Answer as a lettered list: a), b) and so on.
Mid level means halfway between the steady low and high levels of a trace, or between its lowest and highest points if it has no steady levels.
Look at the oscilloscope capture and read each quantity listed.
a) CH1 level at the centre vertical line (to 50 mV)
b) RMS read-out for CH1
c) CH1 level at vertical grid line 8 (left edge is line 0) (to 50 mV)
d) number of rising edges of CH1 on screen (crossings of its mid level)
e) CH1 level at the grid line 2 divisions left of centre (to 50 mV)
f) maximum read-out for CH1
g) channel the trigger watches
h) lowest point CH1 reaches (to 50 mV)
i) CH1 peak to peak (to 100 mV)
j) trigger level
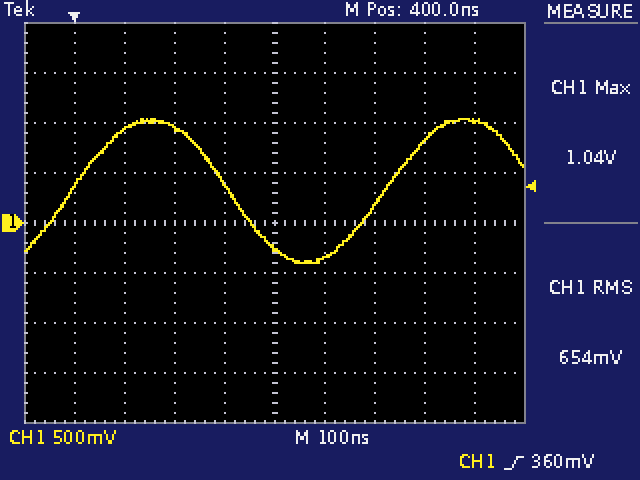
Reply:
a) -250 mV
b) 654 mV
c) 800 mV
d) 2
e) 950 mV
f) 1.04 V
g) CH1
h) -400 mV
i) 1.40 V
j) 360 mV
